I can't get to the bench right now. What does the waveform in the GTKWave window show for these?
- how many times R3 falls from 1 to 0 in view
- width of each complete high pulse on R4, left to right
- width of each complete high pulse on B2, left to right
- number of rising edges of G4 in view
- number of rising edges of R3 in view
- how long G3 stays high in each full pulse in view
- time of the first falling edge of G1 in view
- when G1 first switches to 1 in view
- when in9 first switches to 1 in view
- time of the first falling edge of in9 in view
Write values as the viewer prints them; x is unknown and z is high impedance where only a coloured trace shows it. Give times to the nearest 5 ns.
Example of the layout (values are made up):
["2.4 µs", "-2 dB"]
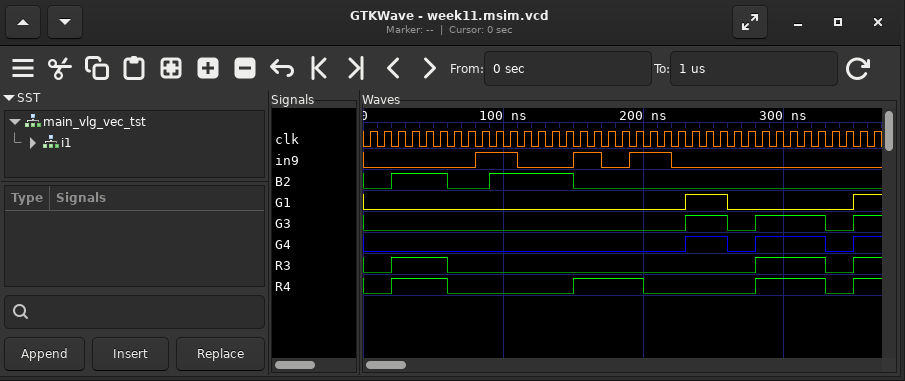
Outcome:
["2", "40 ns, 50 ns, 50 ns", "40 ns, 60 ns", "3", "3", "30 ns, 50 ns", "260 ns", "230 ns", "80 ns", "110 ns"]
